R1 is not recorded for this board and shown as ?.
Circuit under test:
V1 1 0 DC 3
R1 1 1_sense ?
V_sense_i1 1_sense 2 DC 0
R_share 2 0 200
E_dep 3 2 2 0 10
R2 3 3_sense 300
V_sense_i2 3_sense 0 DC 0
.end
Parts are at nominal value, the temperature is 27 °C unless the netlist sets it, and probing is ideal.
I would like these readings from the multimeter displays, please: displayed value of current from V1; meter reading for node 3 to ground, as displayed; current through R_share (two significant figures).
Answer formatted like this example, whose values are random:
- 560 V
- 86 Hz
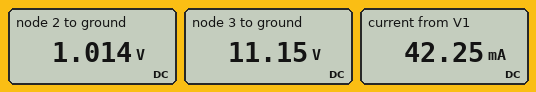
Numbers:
- 42.25 mA
- 11.15 V
- 5.1 mA
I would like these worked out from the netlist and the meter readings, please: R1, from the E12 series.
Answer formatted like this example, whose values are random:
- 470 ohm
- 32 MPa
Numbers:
- 47 Ω
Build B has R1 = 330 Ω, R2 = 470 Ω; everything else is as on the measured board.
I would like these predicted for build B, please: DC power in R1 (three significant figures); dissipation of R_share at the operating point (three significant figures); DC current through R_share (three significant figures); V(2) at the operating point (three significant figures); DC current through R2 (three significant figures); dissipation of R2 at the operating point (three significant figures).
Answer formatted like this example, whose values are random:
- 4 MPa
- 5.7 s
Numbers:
- 22.3 mW
- 418 µW
- 1.45 mA
- 289 mV
- 6.77 mA
- 21.5 mW
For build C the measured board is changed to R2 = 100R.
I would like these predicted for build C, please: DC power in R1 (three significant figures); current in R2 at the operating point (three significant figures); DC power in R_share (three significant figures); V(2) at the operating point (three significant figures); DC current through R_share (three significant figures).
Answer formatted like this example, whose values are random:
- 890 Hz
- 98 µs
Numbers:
- 136 mW
- 51.5 mA
- 1.10 mW
- 468 mV
- 2.34 mA
